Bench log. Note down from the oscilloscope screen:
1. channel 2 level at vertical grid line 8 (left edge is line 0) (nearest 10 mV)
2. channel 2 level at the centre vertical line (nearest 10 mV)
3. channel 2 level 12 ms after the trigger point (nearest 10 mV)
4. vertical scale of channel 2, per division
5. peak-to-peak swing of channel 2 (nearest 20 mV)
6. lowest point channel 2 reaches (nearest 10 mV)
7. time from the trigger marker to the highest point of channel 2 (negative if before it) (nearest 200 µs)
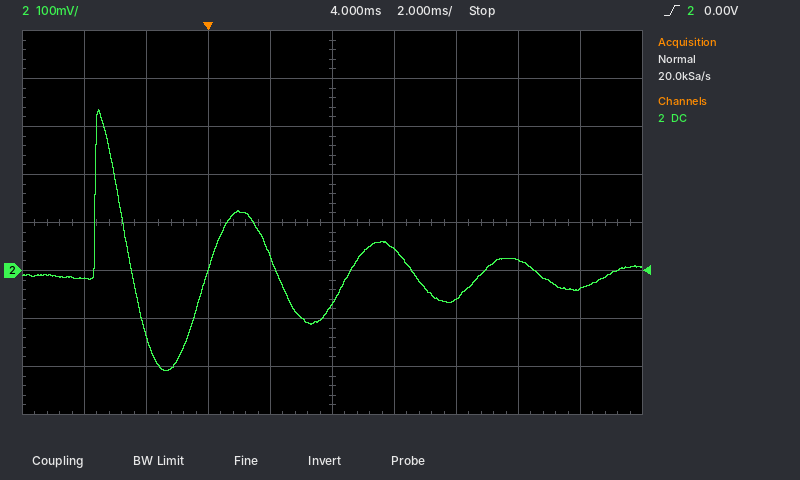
20 mV
-70 mV
-40 mV
100 mV
540 mV
-210 mV
-3.6 ms
